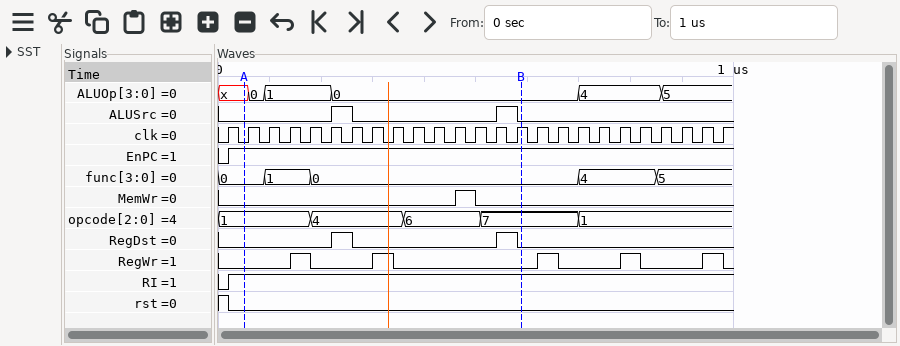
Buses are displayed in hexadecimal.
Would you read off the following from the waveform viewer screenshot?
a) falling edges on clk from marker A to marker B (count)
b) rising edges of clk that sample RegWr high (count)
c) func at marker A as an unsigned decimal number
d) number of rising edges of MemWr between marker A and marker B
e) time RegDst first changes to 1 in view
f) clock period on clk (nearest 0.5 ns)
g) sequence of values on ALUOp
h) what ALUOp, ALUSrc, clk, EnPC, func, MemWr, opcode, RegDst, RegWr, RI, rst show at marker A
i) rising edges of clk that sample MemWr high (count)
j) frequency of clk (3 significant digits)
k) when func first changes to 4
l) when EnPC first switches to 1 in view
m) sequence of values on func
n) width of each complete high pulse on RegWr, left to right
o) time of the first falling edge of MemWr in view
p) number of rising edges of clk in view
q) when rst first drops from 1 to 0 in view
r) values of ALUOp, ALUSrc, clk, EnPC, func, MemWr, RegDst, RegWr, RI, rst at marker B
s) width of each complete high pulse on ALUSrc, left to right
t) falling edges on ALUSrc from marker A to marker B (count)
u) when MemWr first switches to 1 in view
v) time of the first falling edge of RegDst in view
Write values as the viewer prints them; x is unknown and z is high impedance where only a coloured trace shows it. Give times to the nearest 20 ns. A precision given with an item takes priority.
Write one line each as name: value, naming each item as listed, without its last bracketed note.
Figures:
falling edges on clk from marker A to marker B: 13
rising edges of clk that sample RegWr high: 5
func at marker A as an unsigned decimal number: 0
number of rising edges of MemWr between marker A and marker B: 1
time RegDst first changes to 1 in view: 220 ns
clock period on clk: 40 ns
sequence of values on ALUOp: x, 0, 1, 0, 4, 5
what ALUOp, ALUSrc, clk, EnPC, func, MemWr, opcode, RegDst, RegWr, RI, rst show at marker A: ALUOp=x, ALUSrc=0, clk=0, EnPC=1, func=0, MemWr=0, opcode=1, RegDst=0, RegWr=0, RI=1, rst=0
rising edges of clk that sample MemWr high: 1
frequency of clk: 25.0 MHz
when func first changes to 4: 700 ns
when EnPC first switches to 1 in view: 20 ns
sequence of values on func: 0, 1, 0, 4, 5
width of each complete high pulse on RegWr, left to right: 40 ns, 40 ns, 40 ns, 40 ns, 40 ns
time of the first falling edge of MemWr in view: 500 ns
number of rising edges of clk in view: 25
when rst first drops from 1 to 0 in view: 20 ns
values of ALUOp, ALUSrc, clk, EnPC, func, MemWr, RegDst, RegWr, RI, rst at marker B: ALUOp=0, ALUSrc=0, clk=1, EnPC=1, func=0, MemWr=0, RegDst=0, RegWr=0, RI=1, rst=0
width of each complete high pulse on ALUSrc, left to right: 40 ns, 40 ns
falling edges on ALUSrc from marker A to marker B: 2
when MemWr first switches to 1 in view: 460 ns
time of the first falling edge of RegDst in view: 260 ns
